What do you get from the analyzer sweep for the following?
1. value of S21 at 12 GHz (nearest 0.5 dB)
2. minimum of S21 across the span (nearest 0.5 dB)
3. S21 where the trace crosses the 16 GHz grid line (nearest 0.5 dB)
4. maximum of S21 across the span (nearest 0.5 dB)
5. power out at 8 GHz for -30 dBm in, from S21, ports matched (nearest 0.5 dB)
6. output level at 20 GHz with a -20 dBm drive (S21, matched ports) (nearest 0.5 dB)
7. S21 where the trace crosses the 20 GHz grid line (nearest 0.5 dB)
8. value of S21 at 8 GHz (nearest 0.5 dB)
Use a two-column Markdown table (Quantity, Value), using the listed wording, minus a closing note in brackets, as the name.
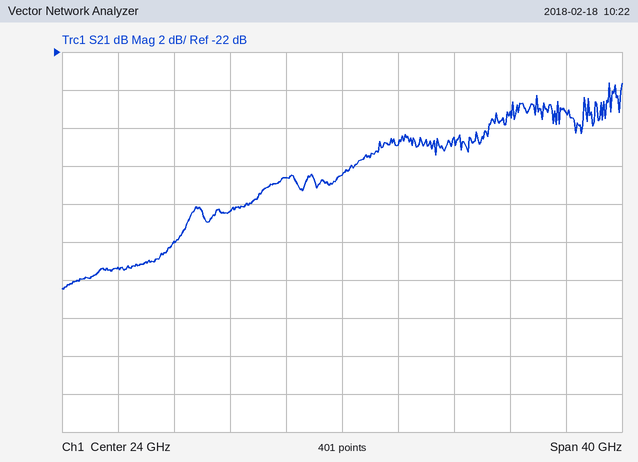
| Quantity | Value |
|---|---|
| value of S21 at 12 GHz | -32.0 dB |
| minimum of S21 across the span | -34.5 dB |
| S21 where the trace crosses the 16 GHz grid line | -30.5 dB |
| maximum of S21 across the span | -23.5 dB |
| power out at 8 GHz for -30 dBm in, from S21, ports matched | -63.5 dBm |
| output level at 20 GHz with a -20 dBm drive (S21, matched ports) | -48.5 dBm |
| S21 where the trace crosses the 20 GHz grid line | -28.5 dB |
| value of S21 at 8 GHz | -33.5 dB |
